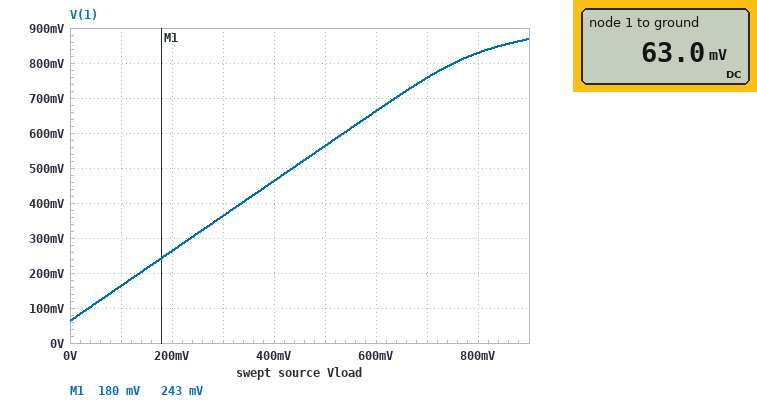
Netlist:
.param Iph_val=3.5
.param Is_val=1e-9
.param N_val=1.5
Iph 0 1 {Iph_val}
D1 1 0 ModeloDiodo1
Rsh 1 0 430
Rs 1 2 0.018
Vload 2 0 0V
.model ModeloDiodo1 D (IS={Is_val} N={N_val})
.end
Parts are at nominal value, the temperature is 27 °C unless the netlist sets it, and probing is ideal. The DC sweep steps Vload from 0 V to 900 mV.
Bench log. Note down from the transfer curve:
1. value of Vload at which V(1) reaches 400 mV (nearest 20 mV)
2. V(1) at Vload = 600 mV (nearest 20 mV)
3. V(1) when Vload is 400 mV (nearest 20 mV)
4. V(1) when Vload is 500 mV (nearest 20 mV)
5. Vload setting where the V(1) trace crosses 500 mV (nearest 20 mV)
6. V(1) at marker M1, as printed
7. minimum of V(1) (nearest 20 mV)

340 mV
660 mV
460 mV
560 mV
440 mV
243 mV
60 mV
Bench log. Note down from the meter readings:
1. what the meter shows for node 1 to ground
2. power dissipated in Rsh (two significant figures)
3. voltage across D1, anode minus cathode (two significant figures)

63.0 mV
9.2 µW
63 mV
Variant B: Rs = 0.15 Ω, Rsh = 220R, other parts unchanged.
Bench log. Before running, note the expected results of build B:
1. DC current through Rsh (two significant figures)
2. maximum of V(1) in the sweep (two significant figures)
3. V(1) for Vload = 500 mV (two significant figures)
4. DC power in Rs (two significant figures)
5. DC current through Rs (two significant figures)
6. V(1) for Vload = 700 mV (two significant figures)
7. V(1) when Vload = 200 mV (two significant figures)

2.4 mA
860 mV
820 mV
1.8 W
3.5 A
840 mV
710 mV
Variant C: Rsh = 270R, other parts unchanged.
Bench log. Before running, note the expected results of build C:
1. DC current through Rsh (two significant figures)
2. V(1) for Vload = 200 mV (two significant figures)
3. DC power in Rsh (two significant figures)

230 µA
260 mV
15 µW
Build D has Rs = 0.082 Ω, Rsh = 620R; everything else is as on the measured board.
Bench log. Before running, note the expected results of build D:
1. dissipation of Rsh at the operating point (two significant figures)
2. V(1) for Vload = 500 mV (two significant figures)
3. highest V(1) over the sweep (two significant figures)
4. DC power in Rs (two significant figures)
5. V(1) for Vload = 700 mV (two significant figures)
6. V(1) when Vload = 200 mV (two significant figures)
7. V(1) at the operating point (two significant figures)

130 µW
760 mV
860 mV
1.0 W
830 mV
490 mV
290 mV
